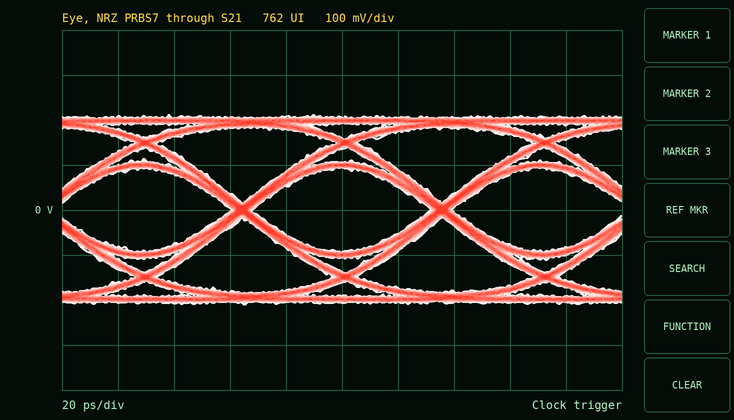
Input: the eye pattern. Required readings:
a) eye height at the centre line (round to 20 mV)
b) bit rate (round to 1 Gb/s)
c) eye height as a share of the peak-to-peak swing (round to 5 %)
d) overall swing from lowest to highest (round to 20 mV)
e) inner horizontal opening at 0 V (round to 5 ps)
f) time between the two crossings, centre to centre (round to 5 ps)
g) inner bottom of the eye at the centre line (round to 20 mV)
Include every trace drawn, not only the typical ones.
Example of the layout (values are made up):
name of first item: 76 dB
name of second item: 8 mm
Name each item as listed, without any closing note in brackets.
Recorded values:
eye height at the centre line: 180 mV
bit rate: 14 Gb/s
eye height as a share of the peak-to-peak swing: 45 %
overall swing from lowest to highest: 420 mV
inner horizontal opening at 0 V: 65 ps
time between the two crossings, centre to centre: 70 ps
inner bottom of the eye at the centre line: -100 mV
